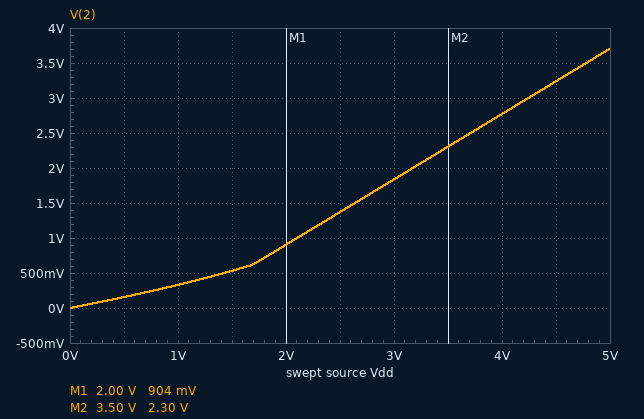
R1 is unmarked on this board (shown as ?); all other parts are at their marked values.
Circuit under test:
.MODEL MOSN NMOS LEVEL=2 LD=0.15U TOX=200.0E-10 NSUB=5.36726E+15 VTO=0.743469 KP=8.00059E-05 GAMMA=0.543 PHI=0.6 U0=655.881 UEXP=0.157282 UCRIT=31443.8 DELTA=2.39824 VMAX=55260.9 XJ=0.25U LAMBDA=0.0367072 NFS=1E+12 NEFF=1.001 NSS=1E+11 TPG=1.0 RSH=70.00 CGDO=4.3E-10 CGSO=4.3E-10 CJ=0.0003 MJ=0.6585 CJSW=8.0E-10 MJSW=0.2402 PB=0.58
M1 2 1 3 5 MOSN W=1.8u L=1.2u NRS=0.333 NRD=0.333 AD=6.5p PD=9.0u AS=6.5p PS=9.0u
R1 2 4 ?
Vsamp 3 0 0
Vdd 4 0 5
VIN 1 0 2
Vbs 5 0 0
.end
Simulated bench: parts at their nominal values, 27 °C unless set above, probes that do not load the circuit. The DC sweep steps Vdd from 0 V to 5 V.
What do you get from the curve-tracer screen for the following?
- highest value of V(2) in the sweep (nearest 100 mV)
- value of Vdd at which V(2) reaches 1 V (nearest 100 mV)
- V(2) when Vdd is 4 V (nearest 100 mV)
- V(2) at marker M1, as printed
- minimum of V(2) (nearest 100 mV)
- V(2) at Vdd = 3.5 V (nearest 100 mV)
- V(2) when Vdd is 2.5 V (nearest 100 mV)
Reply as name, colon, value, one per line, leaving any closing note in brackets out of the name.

highest value of V(2) in the sweep: 3.7 V
value of Vdd at which V(2) reaches 1 V: 2.1 V
V(2) when Vdd is 4 V: 2.8 V
V(2) at marker M1, as printed: 904 mV
minimum of V(2): 0 V
V(2) at Vdd = 3.5 V: 2.3 V
V(2) when Vdd is 2.5 V: 1.4 V
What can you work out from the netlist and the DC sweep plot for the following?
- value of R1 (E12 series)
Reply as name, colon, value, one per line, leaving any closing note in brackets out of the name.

value of R1: 15 kΩ
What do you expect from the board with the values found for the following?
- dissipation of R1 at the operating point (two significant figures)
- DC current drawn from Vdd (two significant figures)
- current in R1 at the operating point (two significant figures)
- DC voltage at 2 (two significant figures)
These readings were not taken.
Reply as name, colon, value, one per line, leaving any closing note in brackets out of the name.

dissipation of R1 at the operating point: 110 µW
DC current drawn from Vdd: 86 µA
current in R1 at the operating point: 86 µA
DC voltage at 2: 3.7 V
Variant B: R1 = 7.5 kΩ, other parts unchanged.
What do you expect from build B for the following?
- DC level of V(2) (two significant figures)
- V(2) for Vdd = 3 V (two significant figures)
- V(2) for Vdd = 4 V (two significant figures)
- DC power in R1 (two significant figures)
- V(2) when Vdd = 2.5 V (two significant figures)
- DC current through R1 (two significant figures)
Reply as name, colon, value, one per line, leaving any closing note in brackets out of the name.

DC level of V(2): 4.3 V
V(2) for Vdd = 3 V: 2.4 V
V(2) for Vdd = 4 V: 3.4 V
DC power in R1: 60 µW
V(2) when Vdd = 2.5 V: 1.9 V
DC current through R1: 89 µA
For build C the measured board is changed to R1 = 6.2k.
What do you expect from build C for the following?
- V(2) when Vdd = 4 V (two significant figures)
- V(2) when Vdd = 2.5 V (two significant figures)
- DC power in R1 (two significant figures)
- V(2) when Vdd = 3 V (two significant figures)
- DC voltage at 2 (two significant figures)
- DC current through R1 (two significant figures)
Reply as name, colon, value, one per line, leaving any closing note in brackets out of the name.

V(2) when Vdd = 4 V: 3.5 V
V(2) when Vdd = 2.5 V: 2.0 V
DC power in R1: 50 µW
V(2) when Vdd = 3 V: 2.5 V
DC voltage at 2: 4.4 V
DC current through R1: 90 µA
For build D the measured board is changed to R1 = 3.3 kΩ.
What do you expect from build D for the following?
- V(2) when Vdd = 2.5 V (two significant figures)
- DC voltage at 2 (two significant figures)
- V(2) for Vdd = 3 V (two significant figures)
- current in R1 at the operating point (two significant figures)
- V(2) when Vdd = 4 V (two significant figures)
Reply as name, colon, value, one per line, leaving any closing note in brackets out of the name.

V(2) when Vdd = 2.5 V: 2.2 V
DC voltage at 2: 4.7 V
V(2) for Vdd = 3 V: 2.7 V
current in R1 at the operating point: 91 µA
V(2) when Vdd = 4 V: 3.7 V
